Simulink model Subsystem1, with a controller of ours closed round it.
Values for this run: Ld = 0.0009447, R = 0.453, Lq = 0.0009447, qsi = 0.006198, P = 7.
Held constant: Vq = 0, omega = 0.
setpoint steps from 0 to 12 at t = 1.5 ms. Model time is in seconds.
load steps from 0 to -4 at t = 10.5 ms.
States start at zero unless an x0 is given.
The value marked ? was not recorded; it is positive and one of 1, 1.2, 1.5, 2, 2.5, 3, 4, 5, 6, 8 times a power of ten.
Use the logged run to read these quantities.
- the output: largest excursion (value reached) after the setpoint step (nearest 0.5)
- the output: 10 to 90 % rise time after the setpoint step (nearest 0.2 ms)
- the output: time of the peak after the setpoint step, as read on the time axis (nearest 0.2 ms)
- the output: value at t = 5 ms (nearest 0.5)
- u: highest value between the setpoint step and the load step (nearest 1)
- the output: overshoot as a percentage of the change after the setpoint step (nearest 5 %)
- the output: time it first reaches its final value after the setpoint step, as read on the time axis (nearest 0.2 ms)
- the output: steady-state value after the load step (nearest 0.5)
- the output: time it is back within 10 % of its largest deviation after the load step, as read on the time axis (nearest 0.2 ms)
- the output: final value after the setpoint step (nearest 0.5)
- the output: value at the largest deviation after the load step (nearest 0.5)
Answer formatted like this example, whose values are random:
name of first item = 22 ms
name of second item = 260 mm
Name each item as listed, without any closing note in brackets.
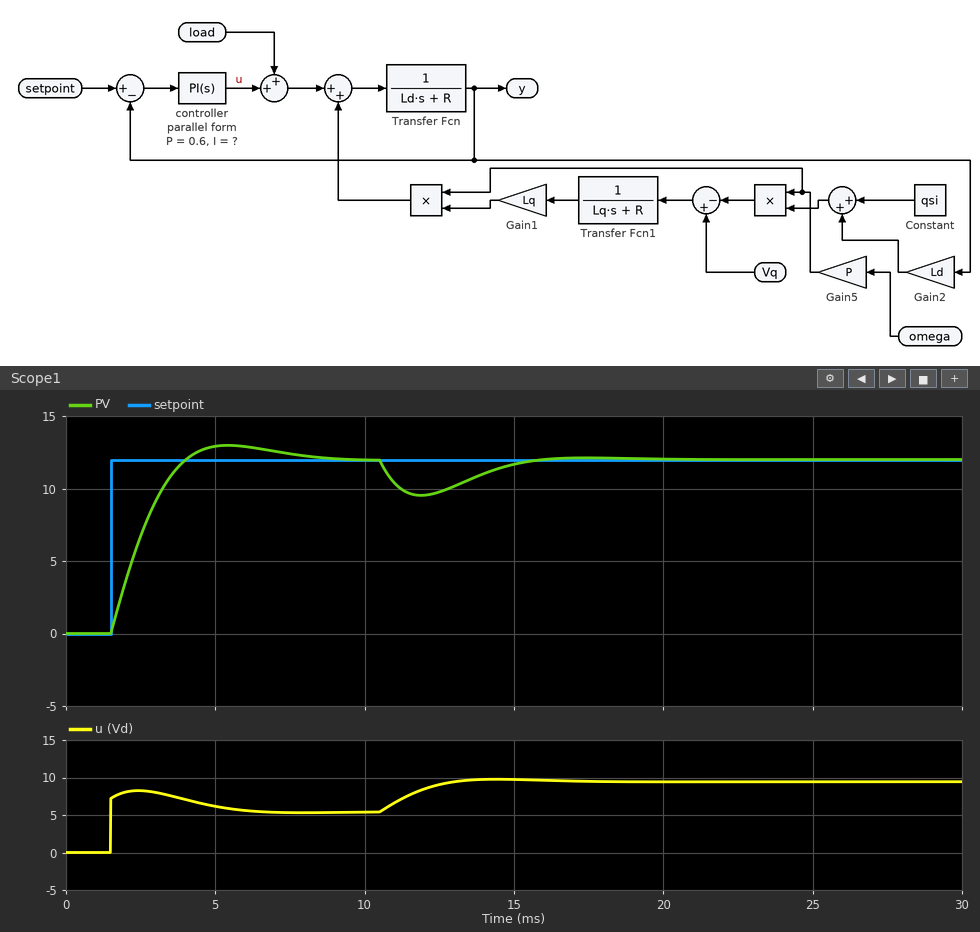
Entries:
the output: largest excursion (value reached) after the setpoint step = 13.0
the output: 10 to 90 % rise time after the setpoint step = 1.8 ms
the output: time of the peak after the setpoint step, as read on the time axis = 5.4 ms
the output: value at t = 5 ms = 13.0
u: highest value between the setpoint step and the load step = 8
the output: overshoot as a percentage of the change after the setpoint step = 10 %
the output: time it first reaches its final value after the setpoint step, as read on the time axis = 4.0 ms
the output: steady-state value after the load step = 12.0
the output: time it is back within 10 % of its largest deviation after the load step, as read on the time axis = 15.2 ms
the output: final value after the setpoint step = 12.0
the output: value at the largest deviation after the load step = 9.5
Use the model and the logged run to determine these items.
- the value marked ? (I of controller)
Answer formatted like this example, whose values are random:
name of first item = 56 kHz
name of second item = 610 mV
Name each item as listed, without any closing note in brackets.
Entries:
the value marked ? = 600
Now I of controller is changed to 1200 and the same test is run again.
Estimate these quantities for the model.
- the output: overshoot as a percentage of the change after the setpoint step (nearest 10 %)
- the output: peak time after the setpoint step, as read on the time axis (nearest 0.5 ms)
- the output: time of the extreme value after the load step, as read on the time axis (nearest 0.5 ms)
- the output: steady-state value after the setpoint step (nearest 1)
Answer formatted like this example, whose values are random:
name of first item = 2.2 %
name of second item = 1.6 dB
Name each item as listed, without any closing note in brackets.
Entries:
the output: overshoot as a percentage of the change after the setpoint step = 20 %
the output: peak time after the setpoint step, as read on the time axis = 4.0 ms
the output: time of the extreme value after the load step, as read on the time axis = 11.5 ms
the output: steady-state value after the setpoint step = 12
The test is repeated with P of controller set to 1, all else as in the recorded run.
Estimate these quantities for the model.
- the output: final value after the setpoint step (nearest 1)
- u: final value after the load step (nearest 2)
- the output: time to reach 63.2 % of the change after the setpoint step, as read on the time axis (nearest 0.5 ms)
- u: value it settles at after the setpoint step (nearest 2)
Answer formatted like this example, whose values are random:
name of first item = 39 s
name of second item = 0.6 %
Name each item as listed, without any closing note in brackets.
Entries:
the output: final value after the setpoint step = 12
u: final value after the load step = 10
the output: time to reach 63.2 % of the change after the setpoint step, as read on the time axis = 2.5 ms
u: value it settles at after the setpoint step = 6
